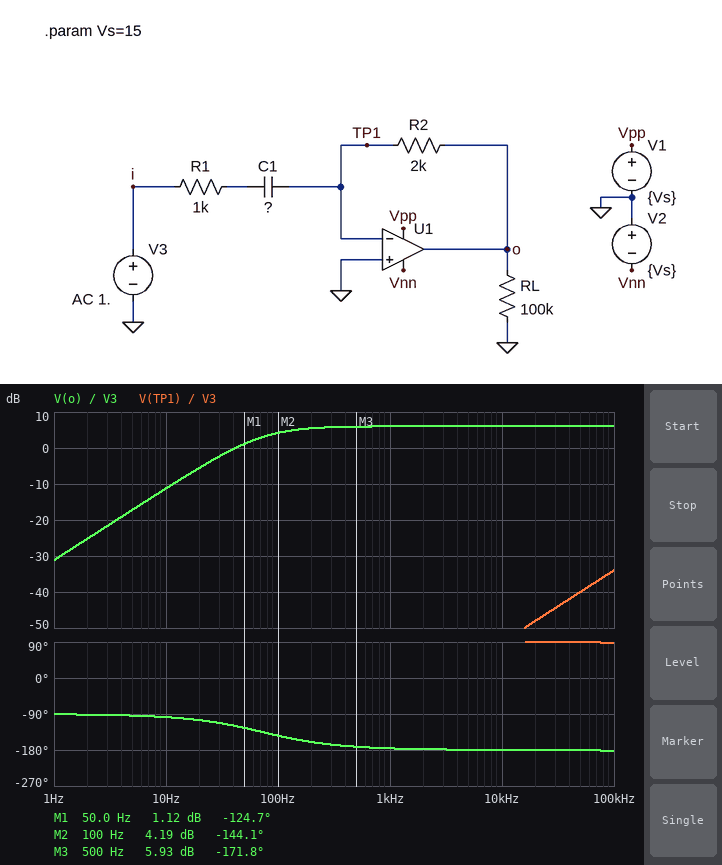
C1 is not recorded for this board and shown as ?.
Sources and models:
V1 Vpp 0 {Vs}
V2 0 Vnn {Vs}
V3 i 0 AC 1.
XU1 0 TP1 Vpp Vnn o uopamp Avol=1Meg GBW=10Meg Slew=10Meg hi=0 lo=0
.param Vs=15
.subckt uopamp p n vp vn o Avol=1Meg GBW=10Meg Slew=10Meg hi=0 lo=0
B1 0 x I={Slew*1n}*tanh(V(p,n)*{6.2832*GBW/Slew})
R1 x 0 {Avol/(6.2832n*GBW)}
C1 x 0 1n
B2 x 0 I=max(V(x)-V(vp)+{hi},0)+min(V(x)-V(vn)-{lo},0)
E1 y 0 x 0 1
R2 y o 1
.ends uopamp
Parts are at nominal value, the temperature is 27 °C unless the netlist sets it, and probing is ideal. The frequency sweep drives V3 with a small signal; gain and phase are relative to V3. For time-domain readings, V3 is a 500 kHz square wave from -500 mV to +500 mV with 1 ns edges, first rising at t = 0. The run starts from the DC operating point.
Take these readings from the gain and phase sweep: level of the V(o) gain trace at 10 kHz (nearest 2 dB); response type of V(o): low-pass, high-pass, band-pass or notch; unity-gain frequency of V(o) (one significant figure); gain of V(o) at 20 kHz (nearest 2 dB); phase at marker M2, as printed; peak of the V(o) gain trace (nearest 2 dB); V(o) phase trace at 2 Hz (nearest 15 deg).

6 dB
high-pass
40 Hz
6 dB
-144.1 deg
6 dB
-90 deg
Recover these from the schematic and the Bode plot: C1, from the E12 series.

2.2 µF
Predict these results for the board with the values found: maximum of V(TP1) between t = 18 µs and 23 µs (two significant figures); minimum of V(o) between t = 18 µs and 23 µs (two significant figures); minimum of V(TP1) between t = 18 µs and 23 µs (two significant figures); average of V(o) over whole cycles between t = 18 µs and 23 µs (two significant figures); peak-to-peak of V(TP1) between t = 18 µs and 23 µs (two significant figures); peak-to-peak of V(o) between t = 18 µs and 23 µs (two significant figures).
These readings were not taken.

660 mV
-2.0 V
-660 mV
-990 mV
1.3 V
2.0 V
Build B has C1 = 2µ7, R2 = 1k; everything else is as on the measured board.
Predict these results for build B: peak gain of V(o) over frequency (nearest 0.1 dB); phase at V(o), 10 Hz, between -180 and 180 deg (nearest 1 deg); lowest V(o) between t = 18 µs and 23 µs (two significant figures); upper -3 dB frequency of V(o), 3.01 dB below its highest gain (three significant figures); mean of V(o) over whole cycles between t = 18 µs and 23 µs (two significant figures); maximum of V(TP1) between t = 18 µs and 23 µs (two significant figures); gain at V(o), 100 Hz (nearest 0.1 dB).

0 dB
-100 deg
-1.0 V
5.00 MHz
-500 mV
500 mV
-1.3 dB
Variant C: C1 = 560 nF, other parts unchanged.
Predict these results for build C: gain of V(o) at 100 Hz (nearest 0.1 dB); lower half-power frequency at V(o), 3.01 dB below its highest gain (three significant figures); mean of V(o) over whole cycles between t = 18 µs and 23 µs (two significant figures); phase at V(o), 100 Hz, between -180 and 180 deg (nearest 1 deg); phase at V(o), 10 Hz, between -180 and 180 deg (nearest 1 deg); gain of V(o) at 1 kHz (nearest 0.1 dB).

-3.6 dB
284 Hz
-960 mV
-109 deg
-92 deg
5.7 dB
